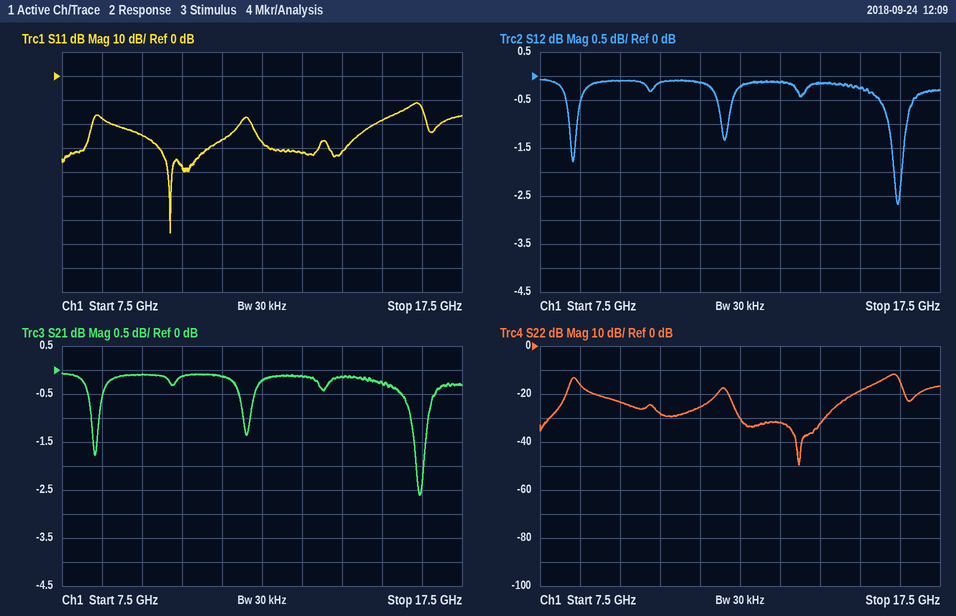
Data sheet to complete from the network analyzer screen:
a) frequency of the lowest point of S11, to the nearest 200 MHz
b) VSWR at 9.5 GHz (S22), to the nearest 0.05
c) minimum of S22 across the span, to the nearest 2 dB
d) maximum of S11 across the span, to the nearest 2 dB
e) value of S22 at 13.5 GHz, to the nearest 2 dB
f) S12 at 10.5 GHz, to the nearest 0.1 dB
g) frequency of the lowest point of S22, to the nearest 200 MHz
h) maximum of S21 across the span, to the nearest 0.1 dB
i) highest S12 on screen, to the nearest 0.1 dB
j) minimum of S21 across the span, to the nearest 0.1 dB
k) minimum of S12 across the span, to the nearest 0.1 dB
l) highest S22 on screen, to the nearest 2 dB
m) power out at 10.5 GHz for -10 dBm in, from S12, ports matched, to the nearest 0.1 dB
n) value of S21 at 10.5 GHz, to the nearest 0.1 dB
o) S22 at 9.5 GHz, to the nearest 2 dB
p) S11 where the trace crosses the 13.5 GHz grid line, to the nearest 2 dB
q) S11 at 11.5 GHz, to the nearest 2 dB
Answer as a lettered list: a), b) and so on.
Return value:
a) 10.2 GHz
b) 1.15
c) -50 dB
d) -12 dB
e) -32 dB
f) -0.1 dB
g) 14.0 GHz
h) -0.1 dB
i) -0.1 dB
j) -2.6 dB
k) -2.7 dB
l) -12 dB
m) -10.1 dBm
n) -0.1 dB
o) -24 dB
p) -32 dB
q) -26 dB
